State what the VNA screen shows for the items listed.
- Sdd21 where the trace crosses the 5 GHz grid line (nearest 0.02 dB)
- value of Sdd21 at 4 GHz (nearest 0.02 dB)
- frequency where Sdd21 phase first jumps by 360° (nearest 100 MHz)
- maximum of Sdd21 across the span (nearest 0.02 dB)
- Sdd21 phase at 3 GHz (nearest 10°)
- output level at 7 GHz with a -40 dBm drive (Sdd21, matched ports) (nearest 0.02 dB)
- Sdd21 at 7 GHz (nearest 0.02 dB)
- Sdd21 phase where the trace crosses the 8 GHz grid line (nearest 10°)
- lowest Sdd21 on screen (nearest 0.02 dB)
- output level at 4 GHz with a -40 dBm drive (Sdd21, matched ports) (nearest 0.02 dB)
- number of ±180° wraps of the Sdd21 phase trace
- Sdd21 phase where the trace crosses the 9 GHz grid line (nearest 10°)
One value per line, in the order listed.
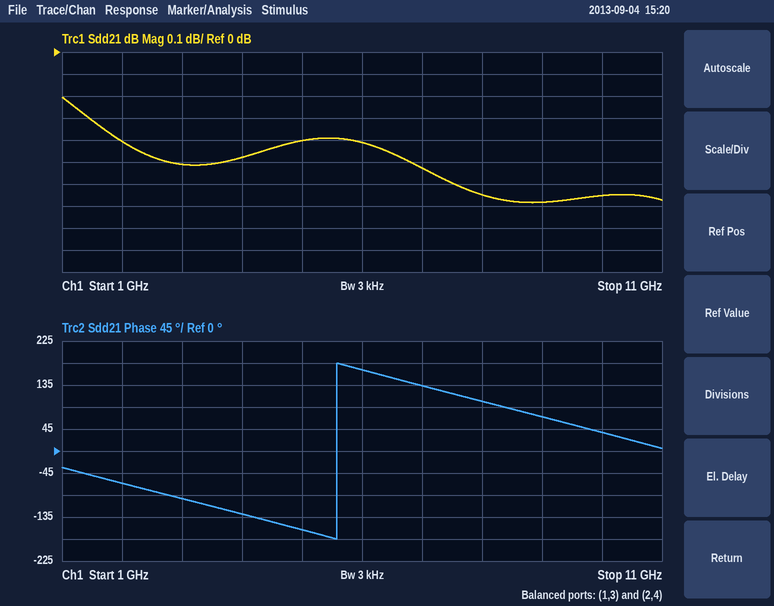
-0.40 dB
-0.48 dB
5.6 GHz
-0.20 dB
-100°
-40.52 dBm
-0.52 dB
100°
-0.68 dB
-40.48 dBm
1
70°
